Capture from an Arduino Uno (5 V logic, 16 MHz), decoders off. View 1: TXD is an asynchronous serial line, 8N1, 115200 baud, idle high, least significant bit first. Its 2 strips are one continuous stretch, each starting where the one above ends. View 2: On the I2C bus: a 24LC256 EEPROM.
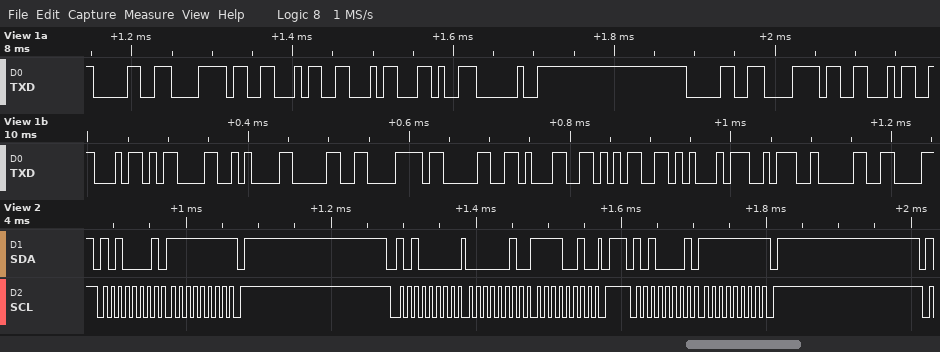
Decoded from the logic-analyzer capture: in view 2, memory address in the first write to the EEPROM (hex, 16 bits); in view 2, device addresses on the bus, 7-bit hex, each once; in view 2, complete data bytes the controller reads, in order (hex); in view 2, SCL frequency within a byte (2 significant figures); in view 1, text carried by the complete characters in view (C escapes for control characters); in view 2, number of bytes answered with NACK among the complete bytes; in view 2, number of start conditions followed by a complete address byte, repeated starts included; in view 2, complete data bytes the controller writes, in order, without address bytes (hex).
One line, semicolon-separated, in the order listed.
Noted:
0x02F2; 0x50; FF FF; 100 kHz; "0xFF, 0xFF\r\n0x015E:0"; 2; 3; 02 F2
